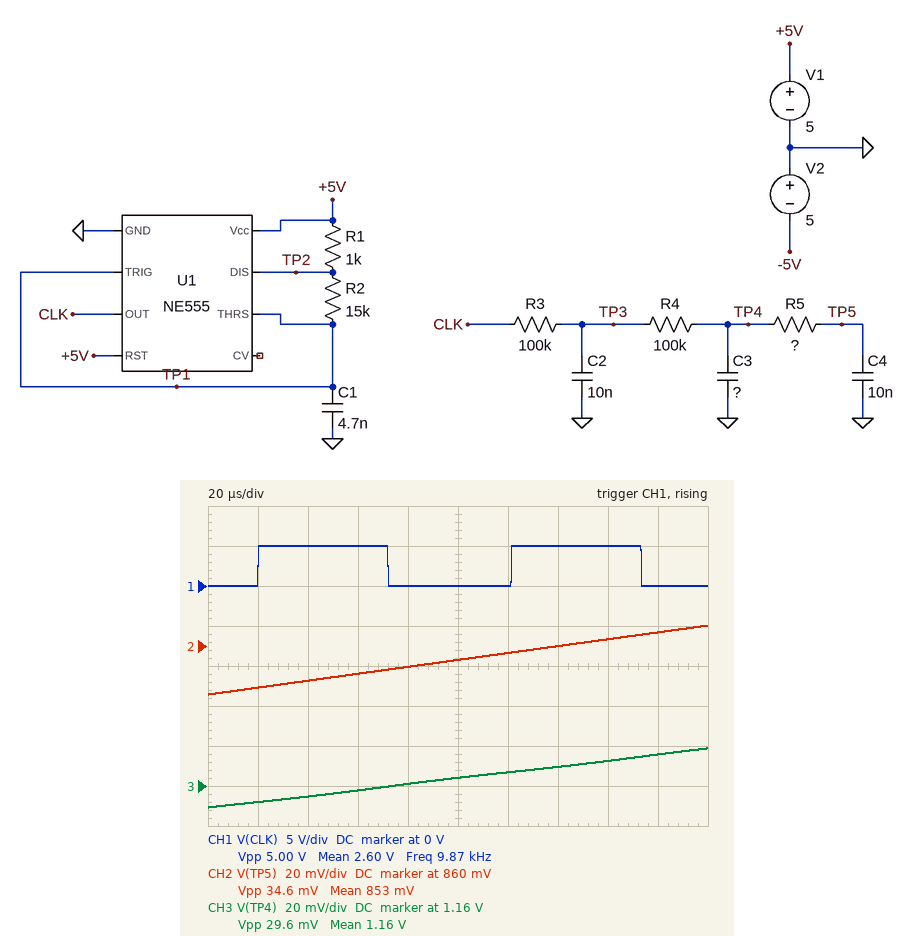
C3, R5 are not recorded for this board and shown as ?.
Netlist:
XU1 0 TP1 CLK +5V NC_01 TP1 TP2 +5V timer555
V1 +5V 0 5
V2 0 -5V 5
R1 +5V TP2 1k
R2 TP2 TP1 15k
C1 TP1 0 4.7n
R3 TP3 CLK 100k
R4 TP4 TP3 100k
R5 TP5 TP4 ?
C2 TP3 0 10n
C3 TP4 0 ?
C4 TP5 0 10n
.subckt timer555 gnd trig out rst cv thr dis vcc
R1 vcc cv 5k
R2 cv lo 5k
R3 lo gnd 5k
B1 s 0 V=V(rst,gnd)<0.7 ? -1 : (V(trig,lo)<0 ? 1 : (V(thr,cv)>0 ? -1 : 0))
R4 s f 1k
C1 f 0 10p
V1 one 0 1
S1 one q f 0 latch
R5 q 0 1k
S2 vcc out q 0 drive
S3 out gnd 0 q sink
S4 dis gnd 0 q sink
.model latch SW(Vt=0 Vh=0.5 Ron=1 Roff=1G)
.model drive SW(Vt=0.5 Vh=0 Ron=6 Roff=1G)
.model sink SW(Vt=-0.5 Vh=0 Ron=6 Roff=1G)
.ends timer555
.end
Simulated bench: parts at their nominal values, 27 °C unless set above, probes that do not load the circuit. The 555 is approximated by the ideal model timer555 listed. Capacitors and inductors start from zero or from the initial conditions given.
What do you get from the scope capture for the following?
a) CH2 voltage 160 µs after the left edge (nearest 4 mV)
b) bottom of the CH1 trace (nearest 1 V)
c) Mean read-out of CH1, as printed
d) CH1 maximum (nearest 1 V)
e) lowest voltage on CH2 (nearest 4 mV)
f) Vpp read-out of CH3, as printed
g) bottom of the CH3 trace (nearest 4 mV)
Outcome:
864 mV
0 V
2.60 V
5 V
836 mV
29.6 mV
1.148 V
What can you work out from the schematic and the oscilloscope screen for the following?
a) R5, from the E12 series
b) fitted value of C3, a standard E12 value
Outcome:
180 kΩ
33 nF
